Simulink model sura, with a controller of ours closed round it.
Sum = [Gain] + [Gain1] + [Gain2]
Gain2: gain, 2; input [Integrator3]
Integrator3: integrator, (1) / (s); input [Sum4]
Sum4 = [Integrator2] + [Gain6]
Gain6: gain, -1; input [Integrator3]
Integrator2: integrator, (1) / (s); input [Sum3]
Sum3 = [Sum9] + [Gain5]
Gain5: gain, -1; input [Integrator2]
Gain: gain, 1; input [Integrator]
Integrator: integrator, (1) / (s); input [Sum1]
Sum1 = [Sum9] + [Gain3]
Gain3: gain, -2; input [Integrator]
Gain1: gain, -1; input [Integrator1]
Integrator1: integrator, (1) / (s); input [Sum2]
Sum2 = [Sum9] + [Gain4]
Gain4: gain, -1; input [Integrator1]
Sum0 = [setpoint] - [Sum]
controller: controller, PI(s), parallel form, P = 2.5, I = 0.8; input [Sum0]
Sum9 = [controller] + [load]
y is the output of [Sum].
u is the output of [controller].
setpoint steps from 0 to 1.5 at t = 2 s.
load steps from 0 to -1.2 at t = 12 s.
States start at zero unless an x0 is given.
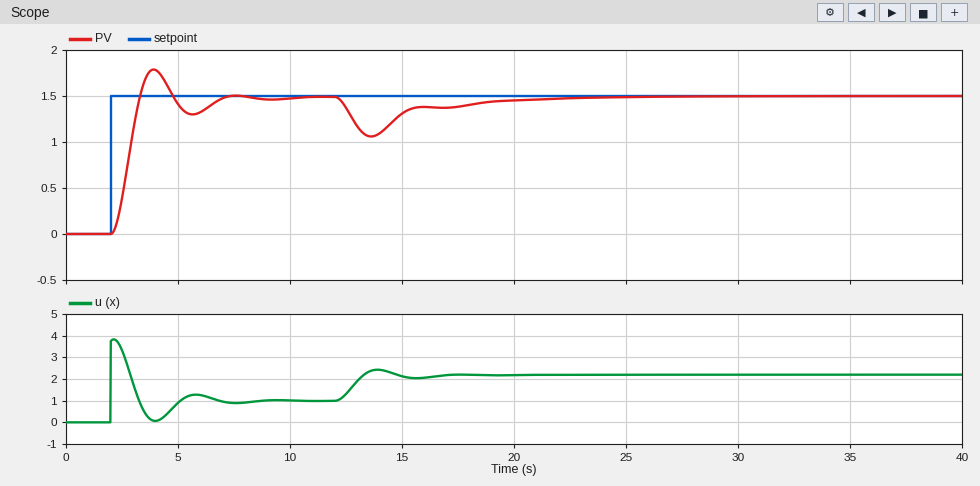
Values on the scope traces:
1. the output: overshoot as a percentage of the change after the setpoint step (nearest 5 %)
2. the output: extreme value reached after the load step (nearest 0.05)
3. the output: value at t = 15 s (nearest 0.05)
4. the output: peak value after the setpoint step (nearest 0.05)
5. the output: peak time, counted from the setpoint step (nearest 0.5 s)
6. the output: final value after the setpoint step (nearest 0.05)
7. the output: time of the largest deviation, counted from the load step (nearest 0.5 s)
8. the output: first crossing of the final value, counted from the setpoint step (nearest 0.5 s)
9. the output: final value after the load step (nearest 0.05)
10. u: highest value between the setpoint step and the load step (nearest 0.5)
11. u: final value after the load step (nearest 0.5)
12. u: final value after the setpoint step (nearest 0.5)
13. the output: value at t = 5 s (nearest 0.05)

20 %
1.05
1.30
1.80
2.0 s
1.50
1.5 s
1.5 s
1.50
4.0
2.0
1.0
1.40
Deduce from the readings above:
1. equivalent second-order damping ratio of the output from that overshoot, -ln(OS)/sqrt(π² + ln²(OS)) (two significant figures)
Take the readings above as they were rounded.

0.46
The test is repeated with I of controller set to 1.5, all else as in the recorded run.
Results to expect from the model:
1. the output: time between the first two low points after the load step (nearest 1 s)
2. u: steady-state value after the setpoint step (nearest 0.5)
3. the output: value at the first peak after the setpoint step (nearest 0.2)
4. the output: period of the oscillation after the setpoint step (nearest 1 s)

4 s
1.0
2.0
4 s
